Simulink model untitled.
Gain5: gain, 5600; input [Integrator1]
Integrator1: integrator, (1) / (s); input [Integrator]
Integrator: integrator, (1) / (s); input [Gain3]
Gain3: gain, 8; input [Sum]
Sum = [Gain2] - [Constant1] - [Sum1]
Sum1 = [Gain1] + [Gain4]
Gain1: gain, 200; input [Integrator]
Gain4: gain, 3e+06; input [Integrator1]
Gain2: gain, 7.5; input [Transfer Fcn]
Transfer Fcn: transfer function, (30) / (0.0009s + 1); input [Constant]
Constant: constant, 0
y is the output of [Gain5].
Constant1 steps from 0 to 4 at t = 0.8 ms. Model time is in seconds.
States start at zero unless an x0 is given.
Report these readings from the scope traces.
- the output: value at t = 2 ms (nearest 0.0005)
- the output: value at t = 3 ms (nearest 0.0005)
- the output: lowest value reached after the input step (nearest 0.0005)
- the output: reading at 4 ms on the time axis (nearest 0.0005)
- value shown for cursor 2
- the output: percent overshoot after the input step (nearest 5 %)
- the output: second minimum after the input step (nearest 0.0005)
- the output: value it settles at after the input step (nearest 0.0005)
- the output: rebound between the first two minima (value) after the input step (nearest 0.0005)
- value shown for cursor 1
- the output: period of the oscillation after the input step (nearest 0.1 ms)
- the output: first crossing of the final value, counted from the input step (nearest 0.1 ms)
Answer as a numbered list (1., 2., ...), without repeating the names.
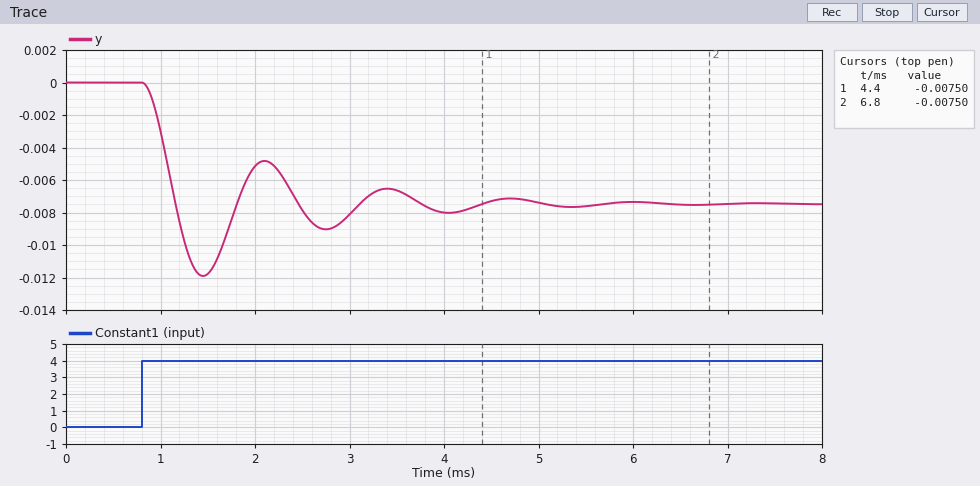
1. -0.0050
2. -0.0080
3. -0.0120
4. -0.0080
5. -0.00750
6. 60 %
7. -0.0090
8. -0.0075
9. -0.0050
10. -0.00750
11. 1.3 ms
12. 0.4 ms
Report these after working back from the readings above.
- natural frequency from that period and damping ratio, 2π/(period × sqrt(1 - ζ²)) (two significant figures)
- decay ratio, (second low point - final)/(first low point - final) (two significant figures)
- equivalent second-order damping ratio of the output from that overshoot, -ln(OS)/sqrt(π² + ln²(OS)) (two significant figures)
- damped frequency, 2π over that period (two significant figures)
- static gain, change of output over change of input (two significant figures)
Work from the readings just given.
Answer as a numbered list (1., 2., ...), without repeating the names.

1. 4.9 rad/ms
2. 0.33
3. 0.16
4. 4.8 rad/ms
5. -0.0019
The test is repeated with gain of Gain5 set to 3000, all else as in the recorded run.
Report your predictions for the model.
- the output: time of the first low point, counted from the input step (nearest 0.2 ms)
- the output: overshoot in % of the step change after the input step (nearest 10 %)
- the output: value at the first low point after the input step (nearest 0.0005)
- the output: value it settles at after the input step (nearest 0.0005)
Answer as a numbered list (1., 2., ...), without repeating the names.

1. 0.6 ms
2. 60 %
3. -0.0065
4. -0.0040
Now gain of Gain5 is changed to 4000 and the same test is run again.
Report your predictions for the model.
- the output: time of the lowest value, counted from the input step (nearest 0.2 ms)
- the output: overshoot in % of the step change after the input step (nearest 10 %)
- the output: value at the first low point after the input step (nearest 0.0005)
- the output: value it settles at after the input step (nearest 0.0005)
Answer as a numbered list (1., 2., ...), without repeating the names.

1. 0.6 ms
2. 60 %
3. -0.0085
4. -0.0055
